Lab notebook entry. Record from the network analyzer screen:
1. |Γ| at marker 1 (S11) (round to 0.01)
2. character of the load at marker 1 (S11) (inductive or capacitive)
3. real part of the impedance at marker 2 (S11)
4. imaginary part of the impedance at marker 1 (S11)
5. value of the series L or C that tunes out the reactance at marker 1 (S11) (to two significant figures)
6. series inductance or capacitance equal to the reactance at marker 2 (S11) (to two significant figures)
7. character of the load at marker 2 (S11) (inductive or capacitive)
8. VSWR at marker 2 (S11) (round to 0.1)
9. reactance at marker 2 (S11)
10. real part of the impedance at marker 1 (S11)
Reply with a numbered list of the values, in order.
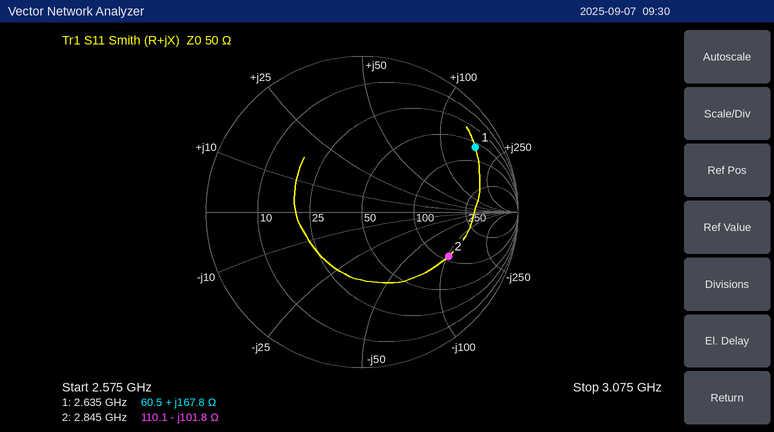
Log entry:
1. 0.84
2. inductive
3. 110.1 Ω
4. +167.8 Ω
5. 360 fF
6. 550 fF
7. capacitive
8. 4.3
9. -101.8 Ω
10. 60.5 Ω
